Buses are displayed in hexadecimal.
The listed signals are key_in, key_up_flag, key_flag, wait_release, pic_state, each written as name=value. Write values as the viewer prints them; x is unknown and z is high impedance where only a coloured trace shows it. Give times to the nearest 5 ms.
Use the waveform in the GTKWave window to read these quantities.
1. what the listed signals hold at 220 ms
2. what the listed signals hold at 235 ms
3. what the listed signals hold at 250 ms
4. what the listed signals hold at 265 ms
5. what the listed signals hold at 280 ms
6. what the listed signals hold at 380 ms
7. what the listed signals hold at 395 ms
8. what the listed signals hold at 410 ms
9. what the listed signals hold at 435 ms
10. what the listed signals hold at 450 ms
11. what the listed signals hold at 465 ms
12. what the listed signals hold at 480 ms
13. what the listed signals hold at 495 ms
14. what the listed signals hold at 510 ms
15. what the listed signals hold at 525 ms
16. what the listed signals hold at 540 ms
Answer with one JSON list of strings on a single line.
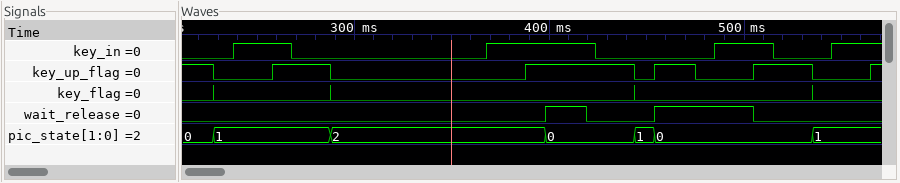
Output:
["key_in=0, key_up_flag=1, key_flag=0, wait_release=0, pic_state=0", "key_in=0, key_up_flag=0, key_flag=0, wait_release=0, pic_state=1", "key_in=1, key_up_flag=0, key_flag=0, wait_release=0, pic_state=1", "key_in=1, key_up_flag=1, key_flag=0, wait_release=0, pic_state=1", "key_in=0, key_up_flag=1, key_flag=0, wait_release=0, pic_state=1", "key_in=1, key_up_flag=0, key_flag=0, wait_release=0, pic_state=2", "key_in=1, key_up_flag=1, key_flag=0, wait_release=0, pic_state=2", "key_in=1, key_up_flag=1, key_flag=0, wait_release=1, pic_state=0", "key_in=0, key_up_flag=1, key_flag=0, wait_release=0, pic_state=0", "key_in=0, key_up_flag=0, key_flag=0, wait_release=0, pic_state=1", "key_in=0, key_up_flag=1, key_flag=0, wait_release=1, pic_state=0", "key_in=0, key_up_flag=0, key_flag=0, wait_release=1, pic_state=0", "key_in=1, key_up_flag=0, key_flag=0, wait_release=1, pic_state=0", "key_in=1, key_up_flag=1, key_flag=0, wait_release=0, pic_state=0", "key_in=0, key_up_flag=1, key_flag=0, wait_release=0, pic_state=0", "key_in=0, key_up_flag=0, key_flag=0, wait_release=0, pic_state=1"]
